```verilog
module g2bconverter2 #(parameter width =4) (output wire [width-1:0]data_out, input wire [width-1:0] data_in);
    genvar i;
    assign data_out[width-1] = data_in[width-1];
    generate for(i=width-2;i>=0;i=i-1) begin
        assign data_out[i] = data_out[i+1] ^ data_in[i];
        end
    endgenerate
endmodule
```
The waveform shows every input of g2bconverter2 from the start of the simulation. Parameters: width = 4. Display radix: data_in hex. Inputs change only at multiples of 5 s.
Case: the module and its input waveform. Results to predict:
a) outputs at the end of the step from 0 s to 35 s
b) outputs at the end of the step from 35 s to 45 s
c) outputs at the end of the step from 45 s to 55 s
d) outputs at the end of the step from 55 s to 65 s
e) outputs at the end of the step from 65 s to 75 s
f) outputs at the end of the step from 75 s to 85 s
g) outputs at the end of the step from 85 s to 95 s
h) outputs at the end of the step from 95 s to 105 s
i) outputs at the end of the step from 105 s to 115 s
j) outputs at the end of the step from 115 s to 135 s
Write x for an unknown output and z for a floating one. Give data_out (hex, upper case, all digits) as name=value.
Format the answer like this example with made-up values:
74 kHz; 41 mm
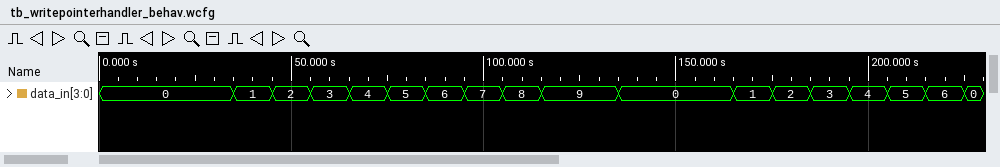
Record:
data_out=0; data_out=1; data_out=3; data_out=2; data_out=7; data_out=6; data_out=4; data_out=5; data_out=F; data_out=E
